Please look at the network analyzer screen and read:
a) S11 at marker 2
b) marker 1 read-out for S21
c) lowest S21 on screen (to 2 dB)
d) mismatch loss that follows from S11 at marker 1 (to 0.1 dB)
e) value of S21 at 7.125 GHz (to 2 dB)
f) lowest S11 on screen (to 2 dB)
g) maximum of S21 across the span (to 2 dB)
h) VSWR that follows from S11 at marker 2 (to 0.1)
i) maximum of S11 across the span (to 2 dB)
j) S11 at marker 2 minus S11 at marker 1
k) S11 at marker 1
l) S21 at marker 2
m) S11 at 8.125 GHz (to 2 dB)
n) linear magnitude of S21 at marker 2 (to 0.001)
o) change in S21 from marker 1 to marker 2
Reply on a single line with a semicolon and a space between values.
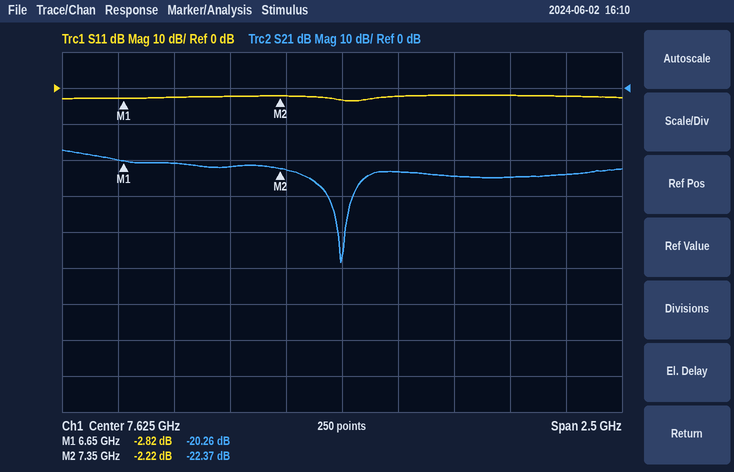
-2.22 dB; -20.26 dB; -48 dB; 3.2 dB; -22 dB; -4 dB; -18 dB; 7.9; -2 dB; 0.60 dB; -2.82 dB; -22.37 dB; -2 dB; 0.076; -2.11 dB
